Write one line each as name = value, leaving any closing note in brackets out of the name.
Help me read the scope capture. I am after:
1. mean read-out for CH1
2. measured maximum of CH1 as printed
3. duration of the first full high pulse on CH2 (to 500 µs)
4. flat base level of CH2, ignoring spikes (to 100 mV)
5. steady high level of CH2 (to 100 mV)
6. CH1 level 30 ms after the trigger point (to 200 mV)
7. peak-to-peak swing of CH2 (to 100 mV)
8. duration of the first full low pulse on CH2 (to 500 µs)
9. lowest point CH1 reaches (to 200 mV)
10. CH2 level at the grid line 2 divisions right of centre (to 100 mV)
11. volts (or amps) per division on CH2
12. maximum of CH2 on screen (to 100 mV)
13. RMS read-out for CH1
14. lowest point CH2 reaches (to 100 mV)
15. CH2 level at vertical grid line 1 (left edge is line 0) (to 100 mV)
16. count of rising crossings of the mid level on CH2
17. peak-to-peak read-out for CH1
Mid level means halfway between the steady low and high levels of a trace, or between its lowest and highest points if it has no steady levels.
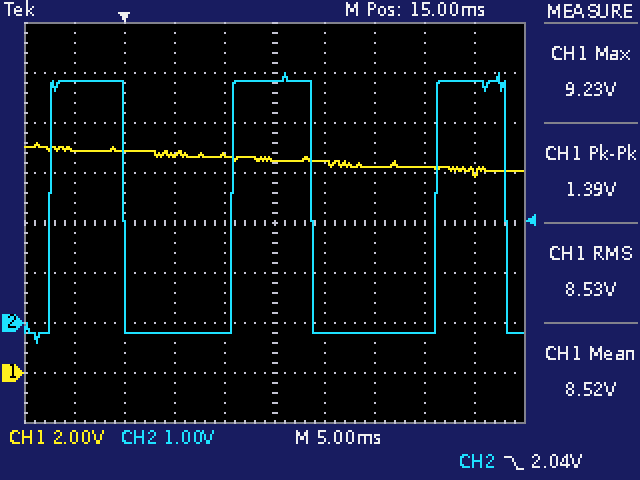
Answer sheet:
mean read-out for CH1 = 8.52 V
measured maximum of CH1 as printed = 9.23 V
duration of the first full high pulse on CH2 = 7.5 ms
flat base level of CH2, ignoring spikes = -200 mV
steady high level of CH2 = 4.8 V
CH1 level 30 ms after the trigger point = 8.2 V
peak-to-peak swing of CH2 = 5.4 V
duration of the first full low pulse on CH2 = 11.0 ms
lowest point CH1 reaches = 7.8 V
CH2 level at the grid line 2 divisions right of centre = -200 mV
volts (or amps) per division on CH2 = 1 V
maximum of CH2 on screen = 5.0 V
RMS read-out for CH1 = 8.53 V
lowest point CH2 reaches = -400 mV
CH2 level at vertical grid line 1 (left edge is line 0) = 4.8 V
count of rising crossings of the mid level on CH2 = 3
peak-to-peak read-out for CH1 = 1.39 V
